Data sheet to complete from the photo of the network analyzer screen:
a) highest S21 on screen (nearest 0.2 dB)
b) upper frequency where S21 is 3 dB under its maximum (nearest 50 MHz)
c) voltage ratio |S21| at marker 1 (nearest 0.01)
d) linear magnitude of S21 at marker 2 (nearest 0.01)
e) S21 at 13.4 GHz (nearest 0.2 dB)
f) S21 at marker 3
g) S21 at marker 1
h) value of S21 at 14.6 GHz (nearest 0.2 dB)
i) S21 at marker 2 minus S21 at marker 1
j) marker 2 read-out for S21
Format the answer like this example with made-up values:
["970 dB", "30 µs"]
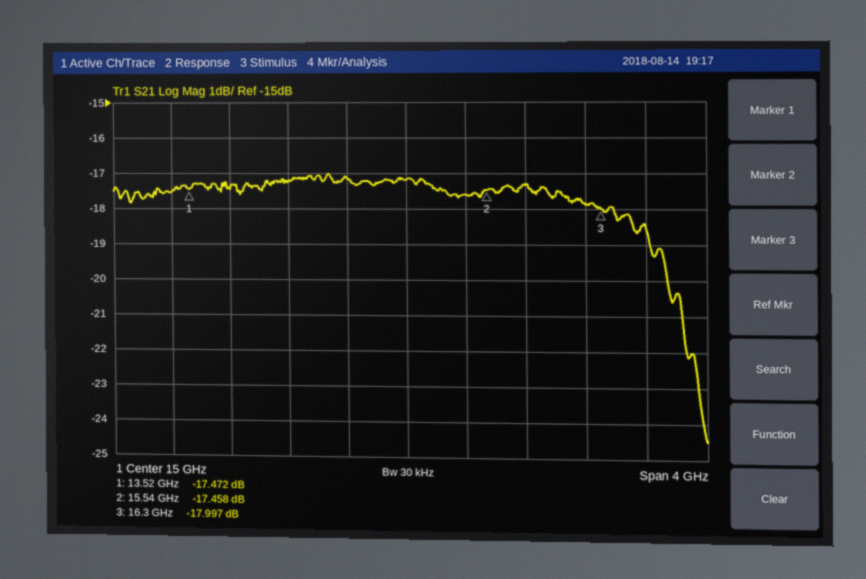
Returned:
["-17.0 dB", "16.75 GHz", "0.13", "0.13", "-17.6 dB", "-17.997 dB", "-17.472 dB", "-17.2 dB", "0.014 dB", "-17.458 dB"]
